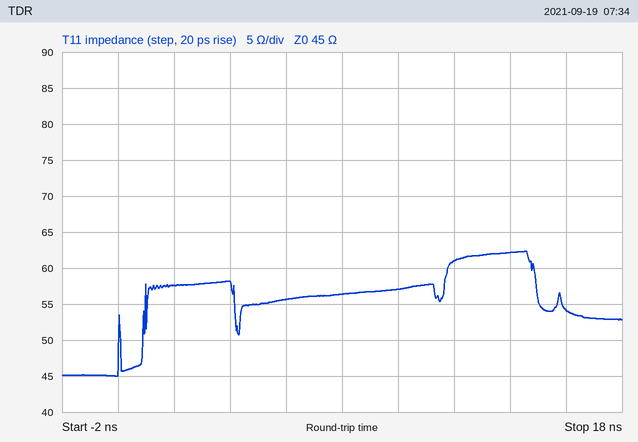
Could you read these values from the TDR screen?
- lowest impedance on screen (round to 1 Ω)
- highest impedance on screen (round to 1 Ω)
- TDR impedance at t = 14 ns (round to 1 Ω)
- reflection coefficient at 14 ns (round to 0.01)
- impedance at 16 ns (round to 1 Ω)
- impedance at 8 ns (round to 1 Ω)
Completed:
45 Ω
62 Ω
62 Ω
+0.16
54 Ω
56 Ω
